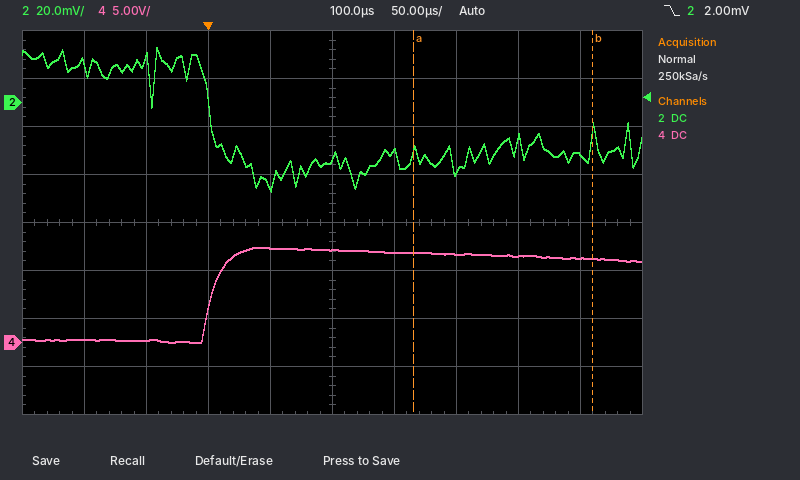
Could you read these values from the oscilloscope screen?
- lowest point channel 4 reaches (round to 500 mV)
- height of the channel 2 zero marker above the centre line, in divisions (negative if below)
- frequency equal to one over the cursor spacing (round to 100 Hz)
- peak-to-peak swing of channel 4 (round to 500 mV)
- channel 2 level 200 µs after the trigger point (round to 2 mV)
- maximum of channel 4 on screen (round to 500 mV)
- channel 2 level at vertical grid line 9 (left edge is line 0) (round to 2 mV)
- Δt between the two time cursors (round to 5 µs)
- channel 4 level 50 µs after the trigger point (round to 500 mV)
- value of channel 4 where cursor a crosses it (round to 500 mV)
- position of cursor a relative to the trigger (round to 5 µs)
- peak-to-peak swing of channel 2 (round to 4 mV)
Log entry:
0.0 V
+2.5 div
6.9 kHz
10.0 V
-28 mV
10.0 V
-22 mV
145 µs
10.0 V
9.5 V
+165 µs
60 mV
